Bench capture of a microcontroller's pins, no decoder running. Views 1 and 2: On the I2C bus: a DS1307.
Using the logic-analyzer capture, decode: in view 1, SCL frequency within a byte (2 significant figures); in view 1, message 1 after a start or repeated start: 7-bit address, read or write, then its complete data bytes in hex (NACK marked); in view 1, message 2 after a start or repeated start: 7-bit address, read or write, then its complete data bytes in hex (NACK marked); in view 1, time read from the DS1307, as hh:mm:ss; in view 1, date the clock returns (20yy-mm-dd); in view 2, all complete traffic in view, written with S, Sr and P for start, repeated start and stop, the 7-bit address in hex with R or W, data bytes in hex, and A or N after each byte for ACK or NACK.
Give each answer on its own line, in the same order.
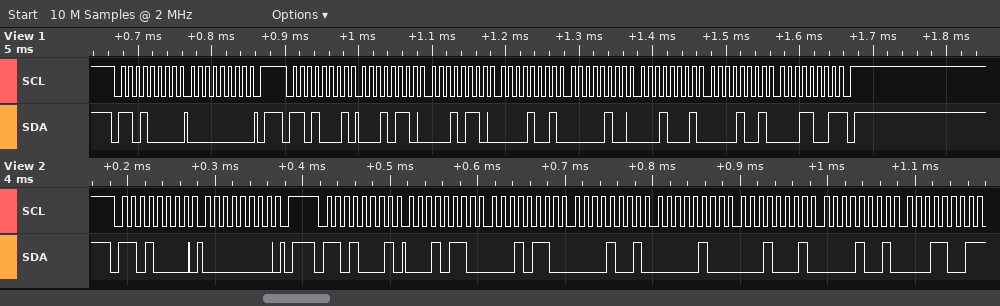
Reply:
100 kHz
0x68 write: 00
0x68 read: 16 16 09 04 11 09 19 NACK
09:16:16
2019-09-11
S 68W A 00 A P S 68R A 16 A 16 A 09 A 04 A 11 A 09 A 19 N
